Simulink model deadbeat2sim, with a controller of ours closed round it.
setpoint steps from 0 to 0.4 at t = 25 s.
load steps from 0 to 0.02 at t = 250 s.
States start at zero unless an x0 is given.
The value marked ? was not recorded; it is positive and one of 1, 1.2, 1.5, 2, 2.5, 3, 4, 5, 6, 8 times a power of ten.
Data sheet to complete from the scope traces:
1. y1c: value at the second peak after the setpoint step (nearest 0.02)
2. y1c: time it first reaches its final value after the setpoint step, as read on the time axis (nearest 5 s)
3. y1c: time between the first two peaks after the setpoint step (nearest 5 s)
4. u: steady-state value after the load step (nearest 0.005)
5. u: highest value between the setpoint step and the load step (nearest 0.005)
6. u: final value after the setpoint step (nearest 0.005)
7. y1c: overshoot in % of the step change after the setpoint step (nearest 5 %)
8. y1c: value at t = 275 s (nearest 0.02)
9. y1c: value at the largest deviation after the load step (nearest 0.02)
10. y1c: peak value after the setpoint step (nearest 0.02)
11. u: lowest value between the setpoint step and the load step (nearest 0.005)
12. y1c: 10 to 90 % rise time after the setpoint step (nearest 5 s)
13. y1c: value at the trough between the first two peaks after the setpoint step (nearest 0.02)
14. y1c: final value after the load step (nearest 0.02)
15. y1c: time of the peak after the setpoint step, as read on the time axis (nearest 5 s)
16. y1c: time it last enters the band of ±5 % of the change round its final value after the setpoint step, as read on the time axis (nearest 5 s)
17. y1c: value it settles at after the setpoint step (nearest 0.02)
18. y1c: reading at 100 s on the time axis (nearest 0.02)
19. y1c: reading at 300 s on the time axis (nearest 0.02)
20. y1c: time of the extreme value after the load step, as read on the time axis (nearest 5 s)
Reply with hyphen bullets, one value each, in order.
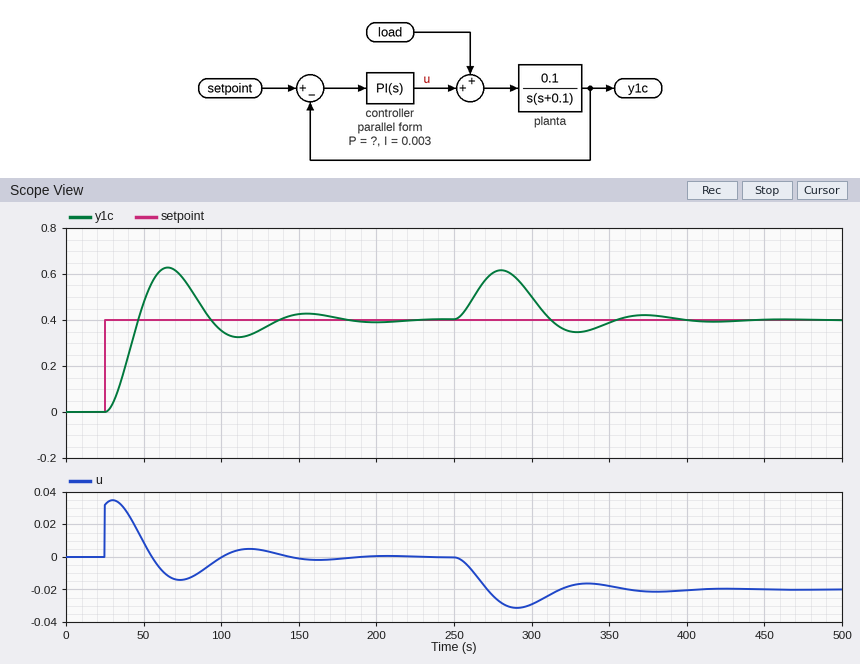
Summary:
- 0.42
- 45 s
- 90 s
- -0.020
- 0.035
- 0.000
- 55 %
- 0.60
- 0.62
- 0.62
- -0.015
- 15 s
- 0.32
- 0.40
- 65 s
- 165 s
- 0.40
- 0.36
- 0.50
- 280 s
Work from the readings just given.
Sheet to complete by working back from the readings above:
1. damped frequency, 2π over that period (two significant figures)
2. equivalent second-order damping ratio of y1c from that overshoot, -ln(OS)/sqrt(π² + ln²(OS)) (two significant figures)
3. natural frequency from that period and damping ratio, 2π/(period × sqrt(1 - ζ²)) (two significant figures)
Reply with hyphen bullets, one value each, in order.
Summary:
- 0.070 rad/s
- 0.19
- 0.071 rad/s
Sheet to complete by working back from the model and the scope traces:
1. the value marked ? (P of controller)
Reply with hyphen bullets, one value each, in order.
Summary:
- 0.08
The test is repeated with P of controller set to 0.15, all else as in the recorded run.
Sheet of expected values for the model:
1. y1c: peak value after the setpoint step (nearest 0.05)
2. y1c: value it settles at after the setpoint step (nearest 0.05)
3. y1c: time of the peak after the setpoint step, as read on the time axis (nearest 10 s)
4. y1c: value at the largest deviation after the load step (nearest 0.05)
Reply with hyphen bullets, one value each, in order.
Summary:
- 0.60
- 0.40
- 50 s
- 0.55
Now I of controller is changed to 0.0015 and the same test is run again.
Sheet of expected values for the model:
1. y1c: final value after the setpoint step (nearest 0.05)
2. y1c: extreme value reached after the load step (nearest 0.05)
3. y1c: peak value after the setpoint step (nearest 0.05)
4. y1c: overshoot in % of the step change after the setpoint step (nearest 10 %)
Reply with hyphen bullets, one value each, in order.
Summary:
- 0.40
- 0.65
- 0.55
- 40 %
